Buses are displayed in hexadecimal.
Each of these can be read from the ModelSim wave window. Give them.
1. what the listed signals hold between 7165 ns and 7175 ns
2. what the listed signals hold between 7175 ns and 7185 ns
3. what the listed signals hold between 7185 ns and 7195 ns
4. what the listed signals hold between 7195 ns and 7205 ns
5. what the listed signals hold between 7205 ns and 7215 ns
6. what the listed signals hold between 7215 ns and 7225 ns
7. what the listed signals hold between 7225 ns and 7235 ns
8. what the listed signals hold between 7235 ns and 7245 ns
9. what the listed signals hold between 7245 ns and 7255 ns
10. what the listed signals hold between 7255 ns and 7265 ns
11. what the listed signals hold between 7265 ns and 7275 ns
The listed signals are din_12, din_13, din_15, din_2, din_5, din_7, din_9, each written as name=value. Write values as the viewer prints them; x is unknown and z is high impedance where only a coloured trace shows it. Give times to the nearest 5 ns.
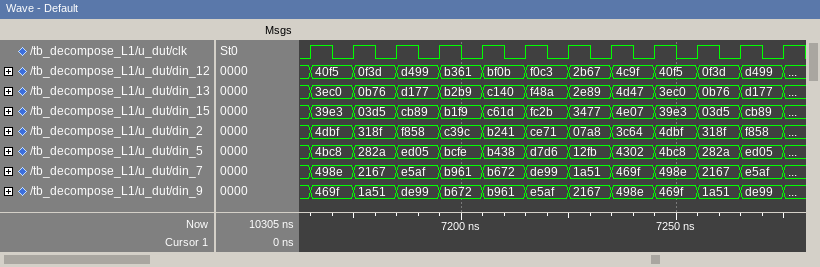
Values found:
din_12=40f5, din_13=3ec0, din_15=39e3, din_2=4dbf, din_5=4bc8, din_7=498e, din_9=469f
din_12=0f3d, din_13=0b76, din_15=03d5, din_2=318f, din_5=282a, din_7=2167, din_9=1a51
din_12=d499, din_13=d177, din_15=cb89, din_2=f858, din_5=ed05, din_7=e5af, din_9=de99
din_12=b361, din_13=b2b9, din_15=b1f9, din_2=c39c, din_5=bcfe, din_7=b961, din_9=b672
din_12=bf0b, din_13=c140, din_15=c61d, din_2=b241, din_5=b438, din_7=b672, din_9=b961
din_12=f0c3, din_13=f48a, din_15=fc2b, din_2=ce71, din_5=d7d6, din_7=de99, din_9=e5af
din_12=2b67, din_13=2e89, din_15=3477, din_2=07a8, din_5=12fb, din_7=1a51, din_9=2167
din_12=4c9f, din_13=4d47, din_15=4e07, din_2=3c64, din_5=4302, din_7=469f, din_9=498e
din_12=40f5, din_13=3ec0, din_15=39e3, din_2=4dbf, din_5=4bc8, din_7=498e, din_9=469f
din_12=0f3d, din_13=0b76, din_15=03d5, din_2=318f, din_5=282a, din_7=2167, din_9=1a51
din_12=d499, din_13=d177, din_15=cb89, din_2=f858, din_5=ed05, din_7=e5af, din_9=de99
